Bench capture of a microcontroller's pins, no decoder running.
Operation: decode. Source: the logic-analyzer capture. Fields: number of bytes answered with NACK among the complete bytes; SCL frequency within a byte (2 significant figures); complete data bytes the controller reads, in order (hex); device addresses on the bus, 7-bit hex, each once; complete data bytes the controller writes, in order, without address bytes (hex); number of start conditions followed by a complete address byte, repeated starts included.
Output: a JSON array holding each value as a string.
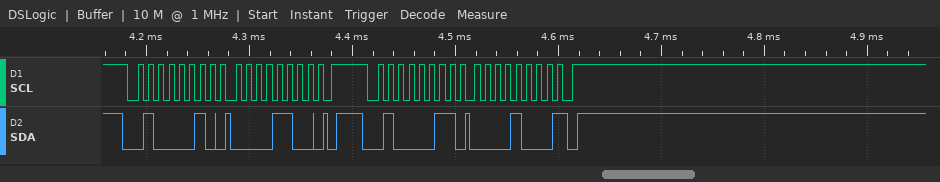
["1", "100 kHz", "08", "0x21", "0C", "2"]
